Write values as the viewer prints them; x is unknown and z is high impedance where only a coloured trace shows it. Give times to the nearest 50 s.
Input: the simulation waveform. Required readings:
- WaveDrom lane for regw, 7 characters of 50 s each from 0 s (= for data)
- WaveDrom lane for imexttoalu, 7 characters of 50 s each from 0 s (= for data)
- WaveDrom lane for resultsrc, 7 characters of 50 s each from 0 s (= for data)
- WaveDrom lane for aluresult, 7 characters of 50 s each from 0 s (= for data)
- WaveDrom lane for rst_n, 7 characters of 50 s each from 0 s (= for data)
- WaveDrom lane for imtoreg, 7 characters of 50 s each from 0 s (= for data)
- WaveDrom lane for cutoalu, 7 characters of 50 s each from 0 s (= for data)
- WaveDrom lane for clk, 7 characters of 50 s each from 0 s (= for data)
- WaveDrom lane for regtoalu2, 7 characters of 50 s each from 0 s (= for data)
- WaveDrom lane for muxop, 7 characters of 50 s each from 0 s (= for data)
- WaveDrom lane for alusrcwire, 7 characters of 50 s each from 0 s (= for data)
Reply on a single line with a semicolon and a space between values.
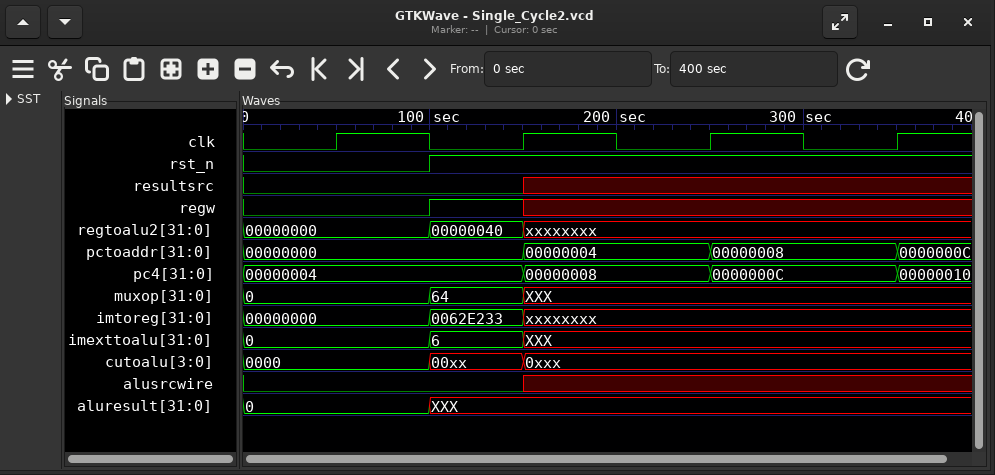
{name: 'regw', wave: '0.1x...'}; {name: 'imexttoalu', wave: '=.=x...', data: '0 6'}; {name: 'resultsrc', wave: '0..x...'}; {name: 'aluresult', wave: '=.x....', data: '0'}; {name: 'rst_n', wave: '0.1....'}; {name: 'imtoreg', wave: '=.=x...', data: '00000000 0062E233'}; {name: 'cutoalu', wave: '=.==...', data: '0000 00xx 0xxx'}; {name: 'clk', wave: '0101010'}; {name: 'regtoalu2', wave: '=.=x...', data: '00000000 00000040'}; {name: 'muxop', wave: '=.=x...', data: '0 64'}; {name: 'alusrcwire', wave: '0..x...'}
